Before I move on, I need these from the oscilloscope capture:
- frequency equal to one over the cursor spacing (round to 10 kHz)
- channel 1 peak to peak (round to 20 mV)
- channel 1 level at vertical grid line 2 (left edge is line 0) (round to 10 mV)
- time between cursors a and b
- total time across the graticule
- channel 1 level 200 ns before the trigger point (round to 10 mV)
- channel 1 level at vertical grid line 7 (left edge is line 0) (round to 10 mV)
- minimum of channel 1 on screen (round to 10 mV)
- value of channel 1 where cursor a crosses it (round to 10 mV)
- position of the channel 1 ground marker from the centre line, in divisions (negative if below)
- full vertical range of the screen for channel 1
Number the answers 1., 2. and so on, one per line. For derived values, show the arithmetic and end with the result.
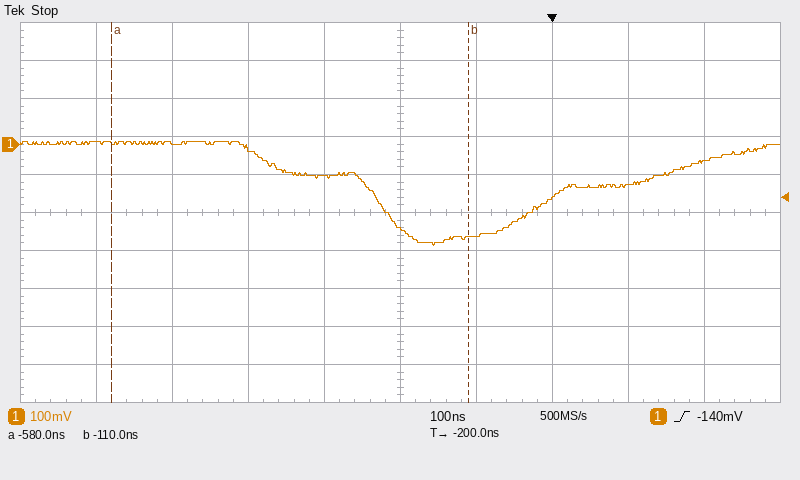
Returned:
1. 1 / 470 ns ≈ 2.13 MHz
2. 280 mV
3. 0 mV
4. -110 ns − (-580 ns) = 470 ns
5. 1 µs
6. -220 mV
7. -140 mV
8. -270 mV
9. 0 mV
10. +1.8 div
11. 1 V
